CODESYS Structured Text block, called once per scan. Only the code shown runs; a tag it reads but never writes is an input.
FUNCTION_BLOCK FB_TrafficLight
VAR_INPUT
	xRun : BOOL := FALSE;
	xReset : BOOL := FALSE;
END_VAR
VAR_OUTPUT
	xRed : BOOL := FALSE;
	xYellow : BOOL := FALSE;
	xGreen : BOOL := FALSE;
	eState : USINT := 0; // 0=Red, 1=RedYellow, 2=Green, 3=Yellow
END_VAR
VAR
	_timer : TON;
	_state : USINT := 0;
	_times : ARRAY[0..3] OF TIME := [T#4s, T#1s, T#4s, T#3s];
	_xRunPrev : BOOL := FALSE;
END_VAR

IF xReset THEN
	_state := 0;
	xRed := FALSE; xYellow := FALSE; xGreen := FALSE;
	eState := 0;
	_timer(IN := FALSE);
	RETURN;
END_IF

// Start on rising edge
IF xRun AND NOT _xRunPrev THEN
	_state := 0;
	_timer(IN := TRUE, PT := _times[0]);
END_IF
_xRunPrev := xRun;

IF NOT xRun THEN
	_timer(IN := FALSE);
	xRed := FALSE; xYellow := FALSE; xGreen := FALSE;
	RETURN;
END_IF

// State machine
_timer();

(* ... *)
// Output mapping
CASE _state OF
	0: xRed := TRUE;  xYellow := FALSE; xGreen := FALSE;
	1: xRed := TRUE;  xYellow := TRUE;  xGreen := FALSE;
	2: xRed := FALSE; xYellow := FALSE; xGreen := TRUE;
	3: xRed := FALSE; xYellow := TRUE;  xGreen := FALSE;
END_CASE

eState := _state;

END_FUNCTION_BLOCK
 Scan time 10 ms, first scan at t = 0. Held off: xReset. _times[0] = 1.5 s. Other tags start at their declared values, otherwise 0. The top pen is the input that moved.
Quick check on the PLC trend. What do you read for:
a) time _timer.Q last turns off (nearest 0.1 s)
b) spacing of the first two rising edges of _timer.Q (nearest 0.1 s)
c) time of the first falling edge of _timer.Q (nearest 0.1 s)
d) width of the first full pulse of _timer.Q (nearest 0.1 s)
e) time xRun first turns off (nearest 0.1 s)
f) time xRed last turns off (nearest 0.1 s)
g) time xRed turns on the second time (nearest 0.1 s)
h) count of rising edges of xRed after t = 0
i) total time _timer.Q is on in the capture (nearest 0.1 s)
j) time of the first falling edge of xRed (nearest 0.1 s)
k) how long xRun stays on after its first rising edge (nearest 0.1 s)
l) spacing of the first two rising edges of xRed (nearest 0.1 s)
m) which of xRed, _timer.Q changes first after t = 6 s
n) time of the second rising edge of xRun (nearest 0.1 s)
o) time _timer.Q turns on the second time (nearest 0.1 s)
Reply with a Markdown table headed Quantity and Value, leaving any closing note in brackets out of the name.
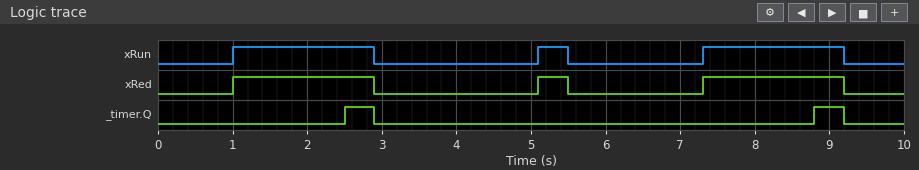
| Quantity | Value |
|---|---|
| time _timer.Q last turns off | 9.2 s |
| spacing of the first two rising edges of _timer.Q | 6.3 s |
| time of the first falling edge of _timer.Q | 2.9 s |
| width of the first full pulse of _timer.Q | 0.4 s |
| time xRun first turns off | 2.9 s |
| time xRed last turns off | 9.2 s |
| time xRed turns on the second time | 5.1 s |
| count of rising edges of xRed after t = 0 | 3 |
| total time _timer.Q is on in the capture | 0.8 s |
| time of the first falling edge of xRed | 2.9 s |
| how long xRun stays on after its first rising edge | 1.9 s |
| spacing of the first two rising edges of xRed | 4.1 s |
| which of xRed, _timer.Q changes first after t = 6 s | xRed |
| time of the second rising edge of xRun | 5.1 s |
| time _timer.Q turns on the second time | 8.8 s |
